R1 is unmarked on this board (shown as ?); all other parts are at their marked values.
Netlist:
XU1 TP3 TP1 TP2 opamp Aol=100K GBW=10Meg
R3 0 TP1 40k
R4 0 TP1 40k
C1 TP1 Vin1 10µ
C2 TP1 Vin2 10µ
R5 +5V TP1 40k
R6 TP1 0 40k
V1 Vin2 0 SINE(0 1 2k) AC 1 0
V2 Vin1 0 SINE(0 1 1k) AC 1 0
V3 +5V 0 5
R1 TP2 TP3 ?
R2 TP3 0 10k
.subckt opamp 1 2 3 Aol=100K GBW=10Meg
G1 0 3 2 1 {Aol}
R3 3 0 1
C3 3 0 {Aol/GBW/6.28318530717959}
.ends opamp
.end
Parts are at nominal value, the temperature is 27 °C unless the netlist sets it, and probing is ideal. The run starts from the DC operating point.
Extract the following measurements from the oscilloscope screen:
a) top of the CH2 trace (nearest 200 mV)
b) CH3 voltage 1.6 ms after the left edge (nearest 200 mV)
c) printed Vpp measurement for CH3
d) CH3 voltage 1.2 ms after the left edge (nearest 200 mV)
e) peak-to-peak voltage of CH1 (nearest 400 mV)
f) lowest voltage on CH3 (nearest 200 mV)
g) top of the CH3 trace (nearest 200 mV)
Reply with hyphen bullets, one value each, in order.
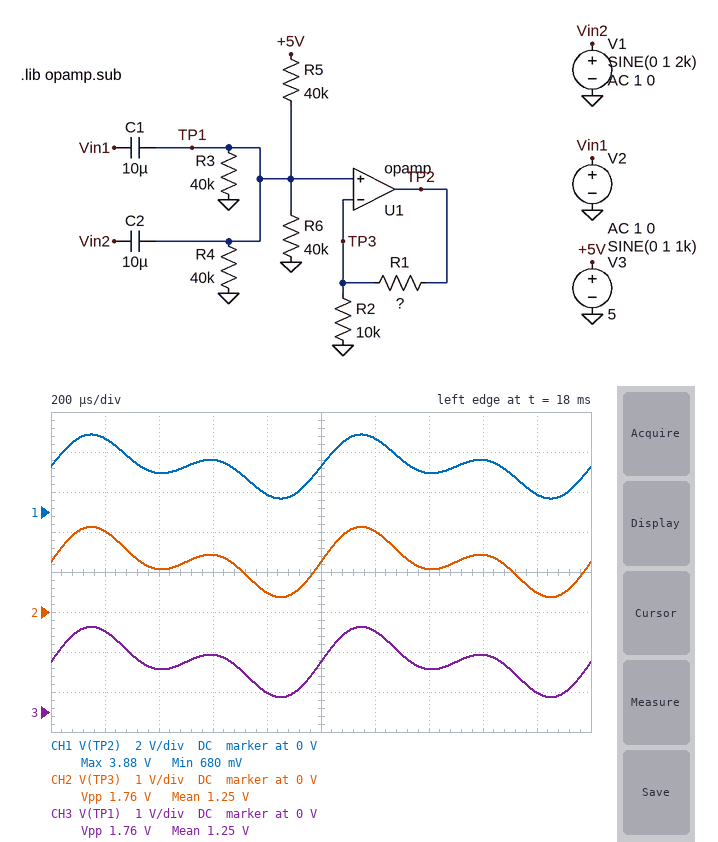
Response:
- 2.2 V
- 1.4 V
- 1.76 V
- 2.0 V
- 3.2 V
- 400 mV
- 2.2 V
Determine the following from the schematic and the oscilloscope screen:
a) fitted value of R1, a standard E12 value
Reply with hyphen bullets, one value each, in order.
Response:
- 8.2 kΩ
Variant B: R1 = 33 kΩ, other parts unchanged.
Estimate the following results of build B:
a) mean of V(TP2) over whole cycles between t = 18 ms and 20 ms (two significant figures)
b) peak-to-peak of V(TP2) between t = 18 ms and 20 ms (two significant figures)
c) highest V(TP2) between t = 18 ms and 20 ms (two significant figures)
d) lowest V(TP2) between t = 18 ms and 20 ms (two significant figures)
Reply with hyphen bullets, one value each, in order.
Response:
- 5.4 V
- 7.6 V
- 9.2 V
- 1.6 V
